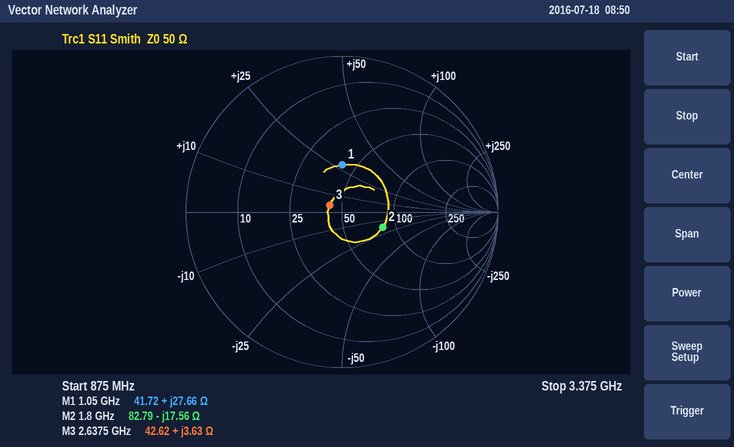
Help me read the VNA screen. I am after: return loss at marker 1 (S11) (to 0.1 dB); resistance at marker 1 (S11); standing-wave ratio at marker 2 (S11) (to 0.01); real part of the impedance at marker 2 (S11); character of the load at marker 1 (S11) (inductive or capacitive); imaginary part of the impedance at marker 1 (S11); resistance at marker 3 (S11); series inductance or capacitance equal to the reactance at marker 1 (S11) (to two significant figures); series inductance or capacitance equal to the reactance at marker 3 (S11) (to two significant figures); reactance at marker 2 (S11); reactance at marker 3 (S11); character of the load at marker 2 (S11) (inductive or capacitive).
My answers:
10.4 dB
41.72 Ω
1.77
82.79 Ω
inductive
+27.66 Ω
42.62 Ω
4.2 nH
220 pH
-17.56 Ω
+3.63 Ω
capacitive
